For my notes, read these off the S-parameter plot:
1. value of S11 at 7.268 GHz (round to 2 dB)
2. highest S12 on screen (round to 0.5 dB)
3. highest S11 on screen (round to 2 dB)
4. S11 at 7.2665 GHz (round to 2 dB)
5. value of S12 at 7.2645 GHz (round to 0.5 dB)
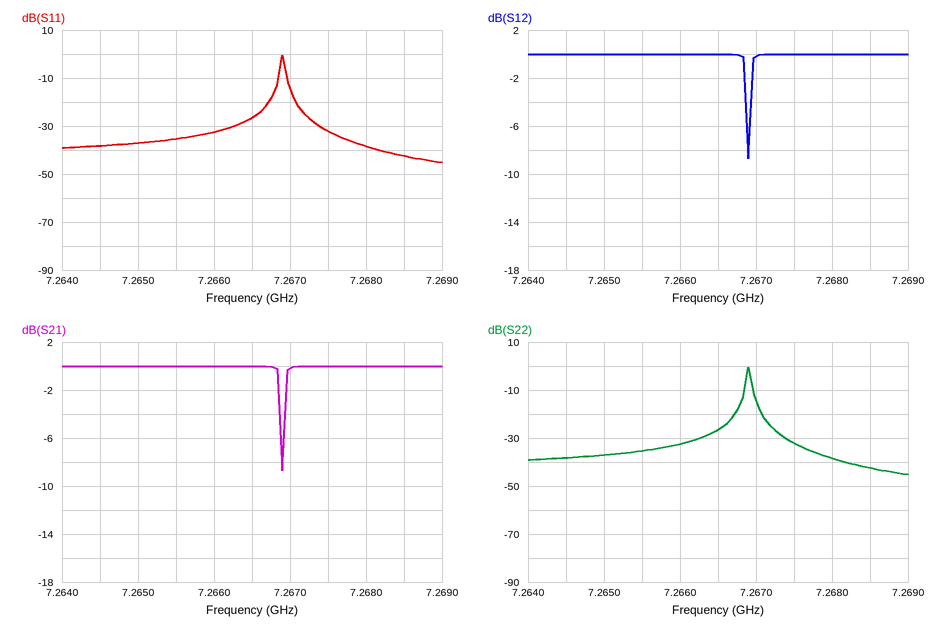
-38 dB
0.0 dB
0 dB
-26 dB
0.0 dB
